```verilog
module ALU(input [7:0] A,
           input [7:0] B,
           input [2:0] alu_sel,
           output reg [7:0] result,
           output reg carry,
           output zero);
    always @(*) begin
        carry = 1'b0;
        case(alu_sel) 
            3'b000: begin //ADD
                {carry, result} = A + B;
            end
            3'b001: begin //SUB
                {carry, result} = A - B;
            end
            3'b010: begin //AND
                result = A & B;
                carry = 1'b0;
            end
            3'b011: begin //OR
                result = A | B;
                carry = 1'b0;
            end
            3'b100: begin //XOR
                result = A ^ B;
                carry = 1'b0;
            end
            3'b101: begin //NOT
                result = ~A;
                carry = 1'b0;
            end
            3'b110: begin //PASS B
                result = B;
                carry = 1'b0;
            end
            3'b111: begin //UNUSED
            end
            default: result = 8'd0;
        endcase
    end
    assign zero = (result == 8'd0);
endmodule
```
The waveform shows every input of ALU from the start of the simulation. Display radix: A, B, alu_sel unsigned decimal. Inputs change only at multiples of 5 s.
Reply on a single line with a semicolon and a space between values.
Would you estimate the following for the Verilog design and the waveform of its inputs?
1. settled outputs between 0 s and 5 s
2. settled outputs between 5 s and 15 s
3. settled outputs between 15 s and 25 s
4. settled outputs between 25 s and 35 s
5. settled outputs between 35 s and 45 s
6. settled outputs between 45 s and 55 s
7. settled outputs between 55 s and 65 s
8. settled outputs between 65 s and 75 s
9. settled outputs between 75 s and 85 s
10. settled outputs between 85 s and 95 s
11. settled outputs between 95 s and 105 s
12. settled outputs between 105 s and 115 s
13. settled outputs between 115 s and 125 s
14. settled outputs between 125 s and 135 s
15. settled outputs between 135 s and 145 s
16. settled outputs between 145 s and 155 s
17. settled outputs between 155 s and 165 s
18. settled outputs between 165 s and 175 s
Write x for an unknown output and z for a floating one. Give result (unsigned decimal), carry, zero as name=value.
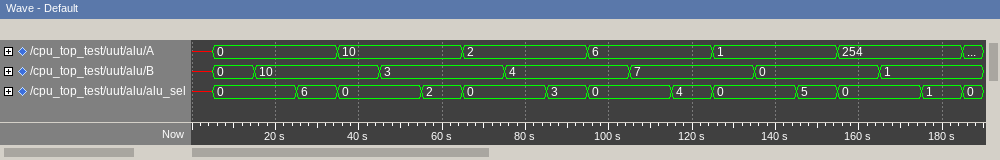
result=x, carry=x, zero=x; result=0, carry=0, zero=1; result=10, carry=0, zero=0; result=10, carry=0, zero=0; result=20, carry=0, zero=0; result=13, carry=0, zero=0; result=2, carry=0, zero=0; result=5, carry=0, zero=0; result=6, carry=0, zero=0; result=6, carry=0, zero=0; result=10, carry=0, zero=0; result=13, carry=0, zero=0; result=1, carry=0, zero=0; result=8, carry=0, zero=0; result=1, carry=0, zero=0; result=254, carry=0, zero=0; result=254, carry=0, zero=0; result=255, carry=0, zero=0
